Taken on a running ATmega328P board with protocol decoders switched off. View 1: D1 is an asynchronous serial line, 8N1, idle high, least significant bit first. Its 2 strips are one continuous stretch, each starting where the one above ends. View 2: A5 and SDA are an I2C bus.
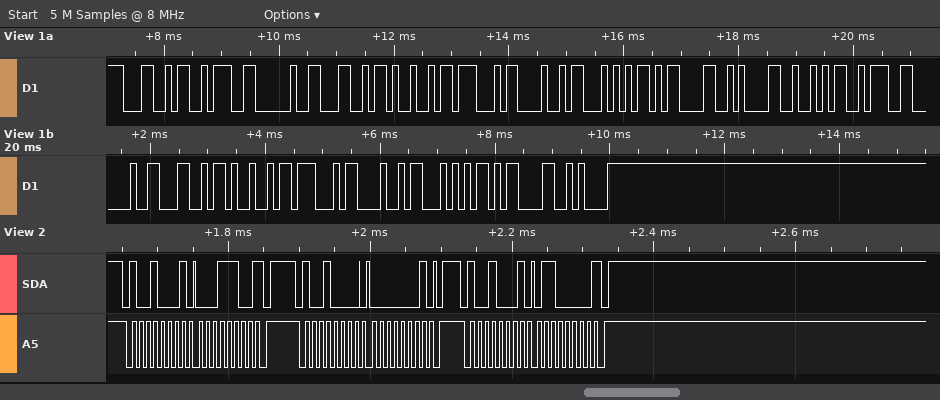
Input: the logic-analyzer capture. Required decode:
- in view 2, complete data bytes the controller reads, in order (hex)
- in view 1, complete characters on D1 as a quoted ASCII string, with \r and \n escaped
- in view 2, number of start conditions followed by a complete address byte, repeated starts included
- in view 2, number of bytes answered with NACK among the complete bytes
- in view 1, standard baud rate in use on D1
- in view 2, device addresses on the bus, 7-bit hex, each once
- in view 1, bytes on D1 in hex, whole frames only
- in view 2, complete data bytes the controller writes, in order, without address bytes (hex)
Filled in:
1C 60
"L: LIGHT\r\nR: LIGHT\r\n"
3
2
9600 baud
0x48
0x4C 0x3A 0x20 0x4C 0x49 0x47 0x48 0x54 0x0D 0x0A 0x52 0x3A 0x20 0x4C 0x49 0x47 0x48 0x54 0x0D 0x0A
01
